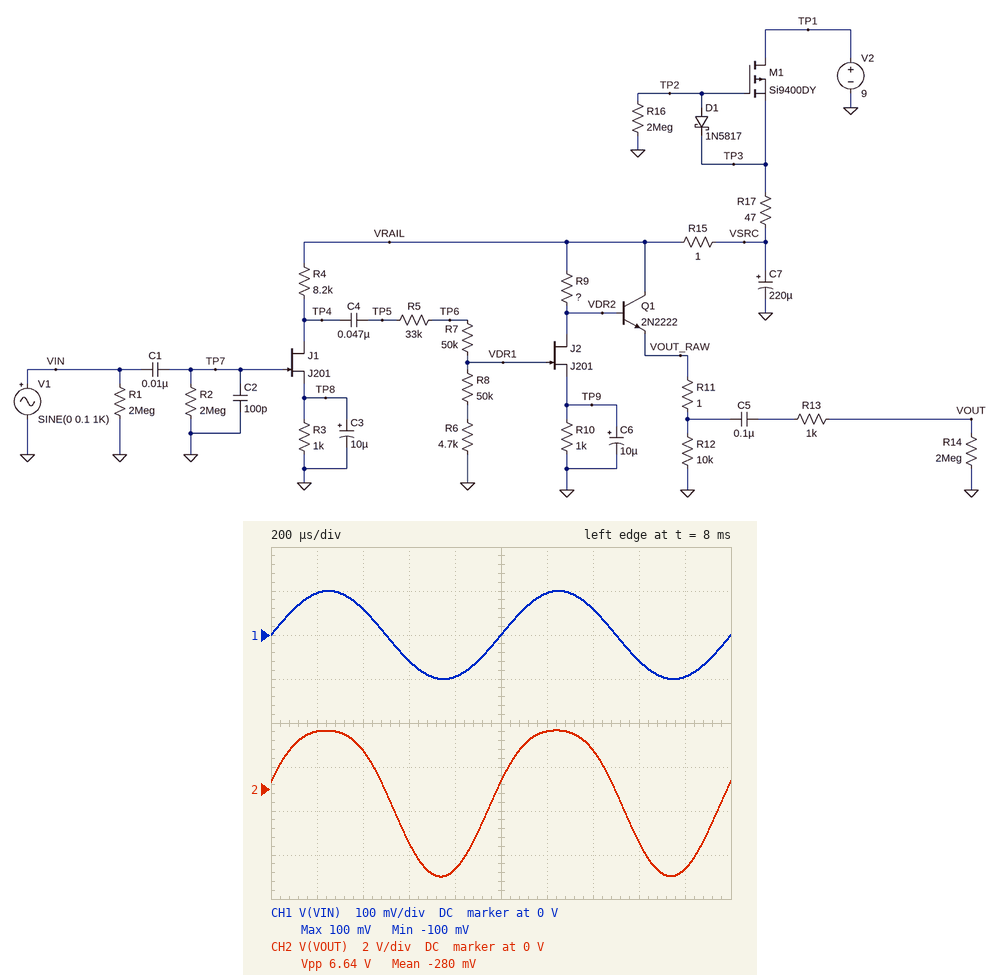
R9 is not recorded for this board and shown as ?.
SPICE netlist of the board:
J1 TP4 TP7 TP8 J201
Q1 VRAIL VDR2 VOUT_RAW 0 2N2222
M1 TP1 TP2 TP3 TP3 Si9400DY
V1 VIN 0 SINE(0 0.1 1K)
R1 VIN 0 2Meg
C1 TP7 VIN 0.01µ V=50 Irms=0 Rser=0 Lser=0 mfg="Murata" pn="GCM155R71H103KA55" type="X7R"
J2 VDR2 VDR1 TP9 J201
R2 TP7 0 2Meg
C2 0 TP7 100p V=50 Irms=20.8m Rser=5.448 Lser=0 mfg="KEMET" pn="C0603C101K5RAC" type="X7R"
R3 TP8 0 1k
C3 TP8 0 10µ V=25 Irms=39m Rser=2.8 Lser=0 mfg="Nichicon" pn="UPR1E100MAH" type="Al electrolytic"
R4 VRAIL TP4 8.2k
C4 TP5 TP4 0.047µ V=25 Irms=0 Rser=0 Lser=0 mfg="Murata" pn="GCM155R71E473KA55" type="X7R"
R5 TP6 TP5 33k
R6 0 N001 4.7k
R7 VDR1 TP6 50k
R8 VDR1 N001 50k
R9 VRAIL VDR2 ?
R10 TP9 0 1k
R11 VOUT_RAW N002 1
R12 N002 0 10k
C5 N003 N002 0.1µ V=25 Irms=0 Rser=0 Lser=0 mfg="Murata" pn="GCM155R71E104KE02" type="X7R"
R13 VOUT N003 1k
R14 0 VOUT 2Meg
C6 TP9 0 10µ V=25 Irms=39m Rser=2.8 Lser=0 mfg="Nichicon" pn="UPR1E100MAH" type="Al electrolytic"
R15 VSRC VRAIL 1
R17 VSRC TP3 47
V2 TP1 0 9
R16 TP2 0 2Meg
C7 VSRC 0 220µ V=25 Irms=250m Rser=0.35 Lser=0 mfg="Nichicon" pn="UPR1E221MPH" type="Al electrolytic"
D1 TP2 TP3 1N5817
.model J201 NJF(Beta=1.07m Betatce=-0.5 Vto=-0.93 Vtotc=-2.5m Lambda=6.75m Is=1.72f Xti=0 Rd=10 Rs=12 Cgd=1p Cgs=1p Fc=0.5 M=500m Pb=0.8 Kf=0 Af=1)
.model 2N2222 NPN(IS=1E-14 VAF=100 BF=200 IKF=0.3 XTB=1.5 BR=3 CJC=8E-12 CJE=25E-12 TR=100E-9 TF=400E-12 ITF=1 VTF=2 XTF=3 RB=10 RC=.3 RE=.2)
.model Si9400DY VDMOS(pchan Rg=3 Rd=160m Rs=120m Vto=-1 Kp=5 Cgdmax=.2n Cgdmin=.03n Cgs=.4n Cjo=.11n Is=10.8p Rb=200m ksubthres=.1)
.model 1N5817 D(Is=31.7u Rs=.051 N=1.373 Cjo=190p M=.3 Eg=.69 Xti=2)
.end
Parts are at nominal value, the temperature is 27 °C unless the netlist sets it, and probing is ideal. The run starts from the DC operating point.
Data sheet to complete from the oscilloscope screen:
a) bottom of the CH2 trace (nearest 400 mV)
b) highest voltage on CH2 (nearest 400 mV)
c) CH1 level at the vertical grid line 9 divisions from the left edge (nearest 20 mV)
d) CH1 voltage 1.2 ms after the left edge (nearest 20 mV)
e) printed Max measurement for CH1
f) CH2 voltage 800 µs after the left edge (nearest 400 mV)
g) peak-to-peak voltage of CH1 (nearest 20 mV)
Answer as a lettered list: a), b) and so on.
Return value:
a) -4.0 V
b) 2.8 V
c) -100 mV
d) 100 mV
e) 100 mV
f) -3.6 V
g) 200 mV
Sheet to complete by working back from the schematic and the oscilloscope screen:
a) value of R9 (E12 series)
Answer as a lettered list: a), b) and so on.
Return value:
a) 8.2 kΩ
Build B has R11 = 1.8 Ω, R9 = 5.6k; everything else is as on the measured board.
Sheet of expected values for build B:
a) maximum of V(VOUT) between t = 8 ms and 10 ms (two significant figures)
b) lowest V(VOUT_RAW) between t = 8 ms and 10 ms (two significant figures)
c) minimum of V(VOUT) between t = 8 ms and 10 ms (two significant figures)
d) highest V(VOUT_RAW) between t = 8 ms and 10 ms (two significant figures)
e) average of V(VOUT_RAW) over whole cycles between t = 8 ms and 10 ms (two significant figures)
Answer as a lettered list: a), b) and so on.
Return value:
a) 1.8 V
b) 3.0 V
c) -2.8 V
d) 7.6 V
e) 5.6 V
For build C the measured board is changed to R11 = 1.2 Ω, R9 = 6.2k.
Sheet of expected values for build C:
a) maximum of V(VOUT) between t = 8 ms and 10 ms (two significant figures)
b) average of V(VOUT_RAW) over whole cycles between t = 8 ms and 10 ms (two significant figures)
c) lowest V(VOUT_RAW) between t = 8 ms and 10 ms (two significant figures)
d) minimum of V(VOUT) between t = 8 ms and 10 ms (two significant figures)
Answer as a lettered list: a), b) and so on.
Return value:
a) 2.0 V
b) 5.4 V
c) 2.5 V
d) -3.1 V
